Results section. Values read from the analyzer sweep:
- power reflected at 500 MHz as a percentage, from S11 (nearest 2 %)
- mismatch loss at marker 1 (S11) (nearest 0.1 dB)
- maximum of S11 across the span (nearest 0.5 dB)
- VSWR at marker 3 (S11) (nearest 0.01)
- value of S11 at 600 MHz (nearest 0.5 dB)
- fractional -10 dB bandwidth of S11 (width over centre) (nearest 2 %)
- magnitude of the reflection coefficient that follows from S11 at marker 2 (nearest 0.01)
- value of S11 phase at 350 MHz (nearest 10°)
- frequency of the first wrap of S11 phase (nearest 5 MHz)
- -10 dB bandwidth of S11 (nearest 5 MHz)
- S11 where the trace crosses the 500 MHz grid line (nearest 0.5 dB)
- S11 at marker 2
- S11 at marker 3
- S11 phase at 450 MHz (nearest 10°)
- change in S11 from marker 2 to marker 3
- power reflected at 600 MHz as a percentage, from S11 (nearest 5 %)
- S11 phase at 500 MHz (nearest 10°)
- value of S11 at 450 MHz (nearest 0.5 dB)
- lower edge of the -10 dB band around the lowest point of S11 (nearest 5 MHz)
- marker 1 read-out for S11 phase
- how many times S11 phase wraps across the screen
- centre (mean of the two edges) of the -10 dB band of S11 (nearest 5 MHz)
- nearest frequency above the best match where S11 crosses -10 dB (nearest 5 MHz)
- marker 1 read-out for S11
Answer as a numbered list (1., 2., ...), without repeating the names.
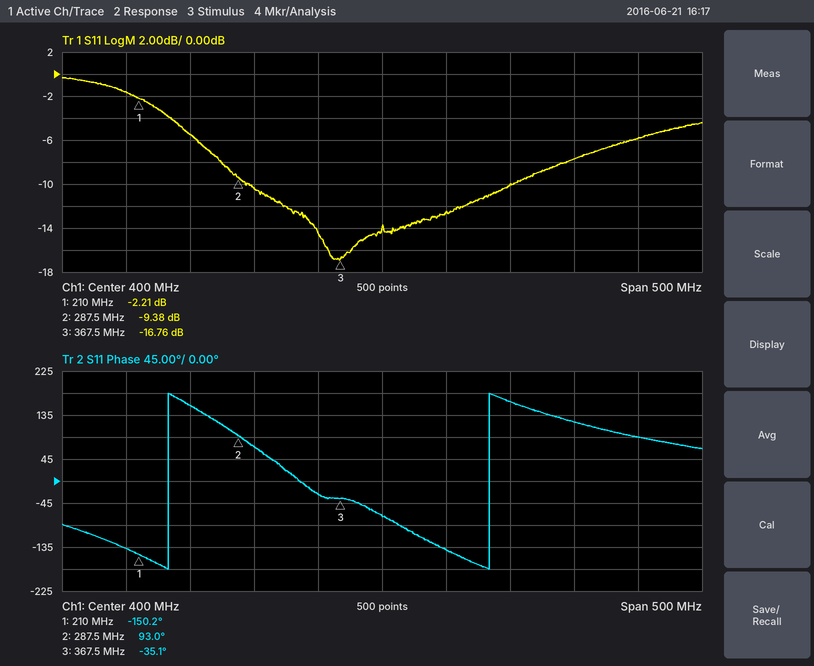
1. 10 %
2. 4.0 dB
3. -0.5 dB
4. 1.34
5. -6.0 dB
6. 52 %
7. 0.34
8. -30°
9. 235 MHz
10. 205 MHz
11. -10.0 dB
12. -9.38 dB
13. -16.76 dB
14. -140°
15. -7.38 dB
16. 25 %
17. 160°
18. -12.5 dB
19. 295 MHz
20. -150.2°
21. 2
22. 400 MHz
23. 500 MHz
24. -2.21 dB
